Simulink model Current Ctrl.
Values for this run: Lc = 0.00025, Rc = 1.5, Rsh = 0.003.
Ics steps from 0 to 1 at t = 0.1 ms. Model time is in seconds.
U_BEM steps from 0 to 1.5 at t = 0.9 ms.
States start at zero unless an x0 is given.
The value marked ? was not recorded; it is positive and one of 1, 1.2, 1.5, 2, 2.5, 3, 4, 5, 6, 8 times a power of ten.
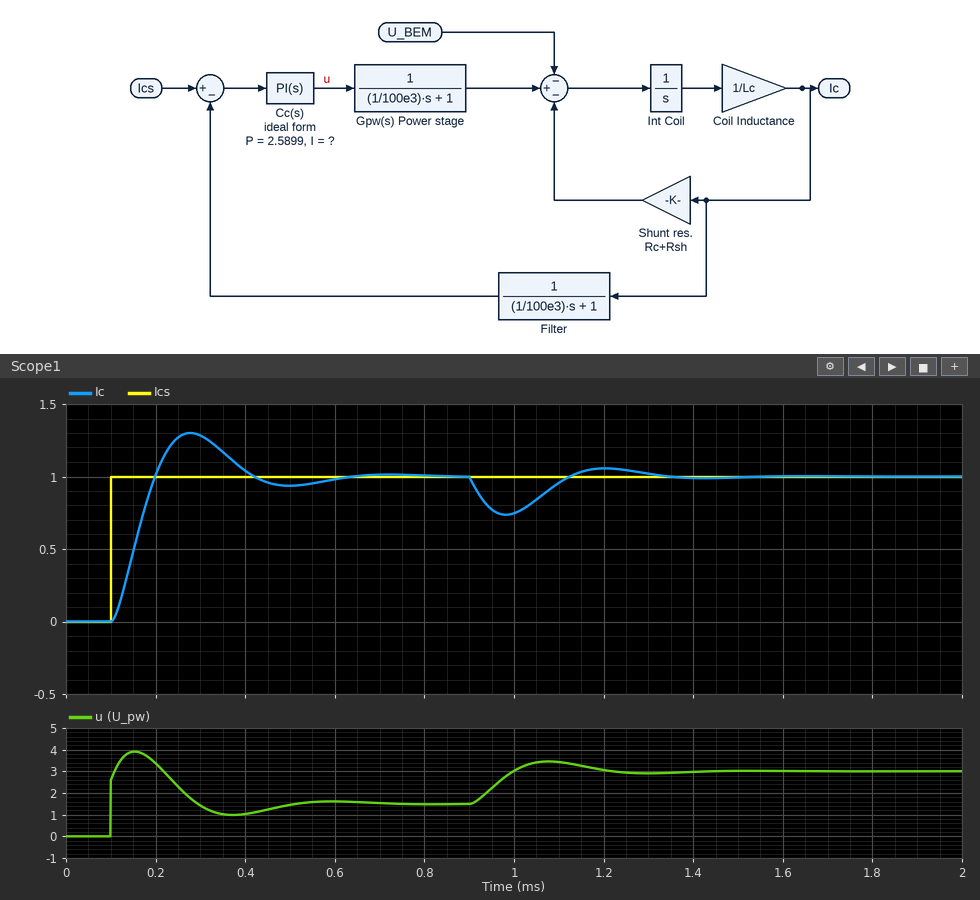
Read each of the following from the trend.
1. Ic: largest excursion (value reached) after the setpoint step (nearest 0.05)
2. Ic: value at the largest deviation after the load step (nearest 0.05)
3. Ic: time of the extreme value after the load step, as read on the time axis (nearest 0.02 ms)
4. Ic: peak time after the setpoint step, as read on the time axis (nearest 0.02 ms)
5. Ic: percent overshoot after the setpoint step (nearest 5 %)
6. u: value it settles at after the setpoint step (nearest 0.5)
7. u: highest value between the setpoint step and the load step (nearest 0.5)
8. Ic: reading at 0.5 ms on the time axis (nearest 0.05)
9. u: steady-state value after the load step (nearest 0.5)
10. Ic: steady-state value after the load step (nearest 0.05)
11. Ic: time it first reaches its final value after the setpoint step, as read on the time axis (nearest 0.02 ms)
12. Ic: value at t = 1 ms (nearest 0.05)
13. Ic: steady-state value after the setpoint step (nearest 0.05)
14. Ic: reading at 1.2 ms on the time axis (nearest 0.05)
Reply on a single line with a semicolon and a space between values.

1.30; 0.75; 0.98 ms; 0.28 ms; 30 %; 1.5; 4.0; 0.95; 3.0; 1.00; 0.20 ms; 0.75; 1.00; 1.05
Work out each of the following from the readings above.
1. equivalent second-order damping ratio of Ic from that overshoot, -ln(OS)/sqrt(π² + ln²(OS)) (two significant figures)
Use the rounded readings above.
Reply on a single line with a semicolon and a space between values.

0.36
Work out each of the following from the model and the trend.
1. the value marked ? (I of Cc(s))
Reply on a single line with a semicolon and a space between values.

20000
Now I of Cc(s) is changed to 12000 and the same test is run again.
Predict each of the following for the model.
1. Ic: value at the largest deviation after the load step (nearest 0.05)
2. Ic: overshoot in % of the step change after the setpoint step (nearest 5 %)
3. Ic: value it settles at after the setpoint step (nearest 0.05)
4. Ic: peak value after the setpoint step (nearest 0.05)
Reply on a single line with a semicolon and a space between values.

0.70; 15 %; 1.00; 1.15
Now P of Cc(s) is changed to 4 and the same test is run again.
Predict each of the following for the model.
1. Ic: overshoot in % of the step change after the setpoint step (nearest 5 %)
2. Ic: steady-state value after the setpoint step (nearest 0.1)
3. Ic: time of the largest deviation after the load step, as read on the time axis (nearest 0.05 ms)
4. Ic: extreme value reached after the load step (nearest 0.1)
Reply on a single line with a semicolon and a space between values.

35 %; 1.0; 0.95 ms; 0.8
